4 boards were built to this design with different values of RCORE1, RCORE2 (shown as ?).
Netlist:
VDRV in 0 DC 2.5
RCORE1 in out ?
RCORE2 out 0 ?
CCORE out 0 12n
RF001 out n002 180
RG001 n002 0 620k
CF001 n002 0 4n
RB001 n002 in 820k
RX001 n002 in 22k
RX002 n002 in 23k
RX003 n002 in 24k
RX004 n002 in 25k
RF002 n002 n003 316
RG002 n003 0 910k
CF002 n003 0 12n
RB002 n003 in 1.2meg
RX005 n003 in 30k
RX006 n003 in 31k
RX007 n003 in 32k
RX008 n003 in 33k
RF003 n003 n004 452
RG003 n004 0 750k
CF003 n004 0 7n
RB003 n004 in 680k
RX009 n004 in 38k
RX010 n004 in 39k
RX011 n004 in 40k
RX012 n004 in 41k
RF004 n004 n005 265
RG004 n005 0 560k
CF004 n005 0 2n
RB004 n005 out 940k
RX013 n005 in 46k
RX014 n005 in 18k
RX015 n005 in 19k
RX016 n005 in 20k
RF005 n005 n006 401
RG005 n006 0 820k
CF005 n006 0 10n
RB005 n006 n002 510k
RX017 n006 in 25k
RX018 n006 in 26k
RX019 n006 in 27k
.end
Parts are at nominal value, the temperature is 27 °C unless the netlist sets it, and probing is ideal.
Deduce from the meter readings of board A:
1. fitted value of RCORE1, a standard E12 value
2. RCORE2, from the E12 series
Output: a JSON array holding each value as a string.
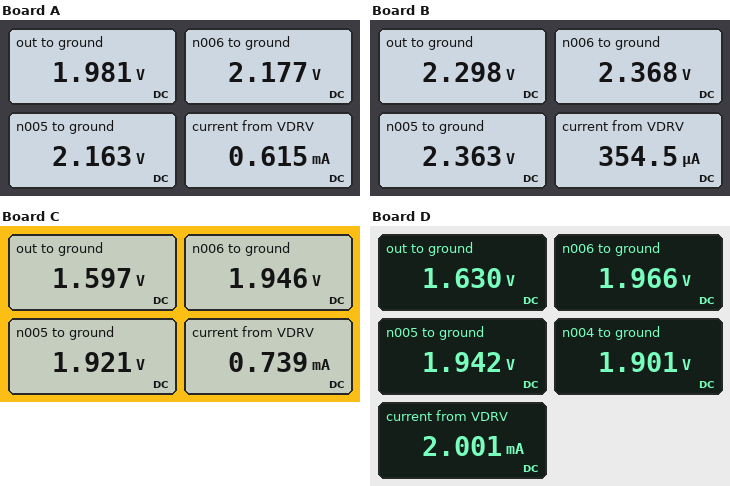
["1.5 kΩ", "3.3 kΩ"]
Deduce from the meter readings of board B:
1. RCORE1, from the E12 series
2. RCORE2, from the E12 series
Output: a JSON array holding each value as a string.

["820 Ω", "6.8 kΩ"]
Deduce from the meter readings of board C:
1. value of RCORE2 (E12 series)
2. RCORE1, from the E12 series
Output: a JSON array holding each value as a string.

["2.2 kΩ", "3.3 kΩ"]
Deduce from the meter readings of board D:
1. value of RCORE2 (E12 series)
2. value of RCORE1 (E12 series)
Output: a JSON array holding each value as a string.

["820 Ω", "560 Ω"]
